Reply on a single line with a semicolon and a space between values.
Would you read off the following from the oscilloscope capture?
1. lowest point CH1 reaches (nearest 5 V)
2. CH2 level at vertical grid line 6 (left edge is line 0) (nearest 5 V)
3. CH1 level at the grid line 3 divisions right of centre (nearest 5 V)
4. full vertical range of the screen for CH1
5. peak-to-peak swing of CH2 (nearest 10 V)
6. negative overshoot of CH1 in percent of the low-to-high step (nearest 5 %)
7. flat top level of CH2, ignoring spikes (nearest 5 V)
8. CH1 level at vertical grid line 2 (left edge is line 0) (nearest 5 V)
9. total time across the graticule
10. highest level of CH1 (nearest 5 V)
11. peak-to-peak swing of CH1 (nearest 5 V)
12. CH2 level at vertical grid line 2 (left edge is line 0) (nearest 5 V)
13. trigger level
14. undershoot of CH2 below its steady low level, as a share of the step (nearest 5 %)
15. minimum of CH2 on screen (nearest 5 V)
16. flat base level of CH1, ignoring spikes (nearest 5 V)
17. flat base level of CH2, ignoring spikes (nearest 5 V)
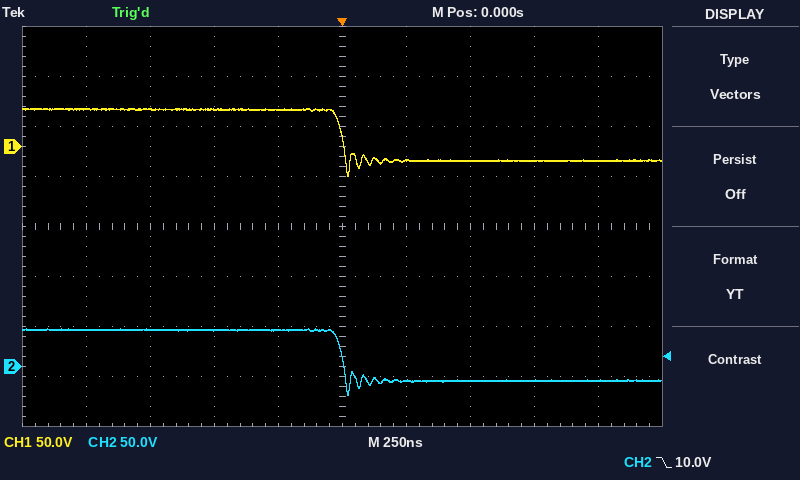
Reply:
-30 V; -15 V; -15 V; 400 V; 70 V; 30 %; 35 V; 35 V; 2.5 µs; 40 V; 70 V; 35 V; 10.0 V; 30 %; -30 V; -15 V; -15 V
